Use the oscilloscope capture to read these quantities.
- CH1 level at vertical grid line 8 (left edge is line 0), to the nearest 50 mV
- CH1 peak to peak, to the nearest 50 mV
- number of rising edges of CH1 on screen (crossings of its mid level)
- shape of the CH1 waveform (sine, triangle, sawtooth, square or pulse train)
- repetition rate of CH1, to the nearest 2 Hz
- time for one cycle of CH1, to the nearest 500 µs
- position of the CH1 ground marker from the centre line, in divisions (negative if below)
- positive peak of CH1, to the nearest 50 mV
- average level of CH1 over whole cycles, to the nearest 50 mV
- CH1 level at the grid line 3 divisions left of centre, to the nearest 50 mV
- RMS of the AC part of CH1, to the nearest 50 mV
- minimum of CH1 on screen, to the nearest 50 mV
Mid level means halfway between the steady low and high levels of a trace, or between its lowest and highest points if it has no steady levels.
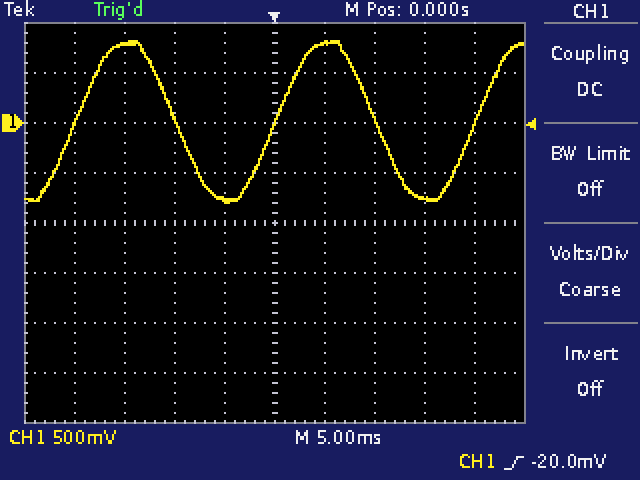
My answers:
-750 mV
1.60 V
3
sine
50 Hz
20.0 ms
+2.0 div
800 mV
0 mV
800 mV
550 mV
-800 mV
